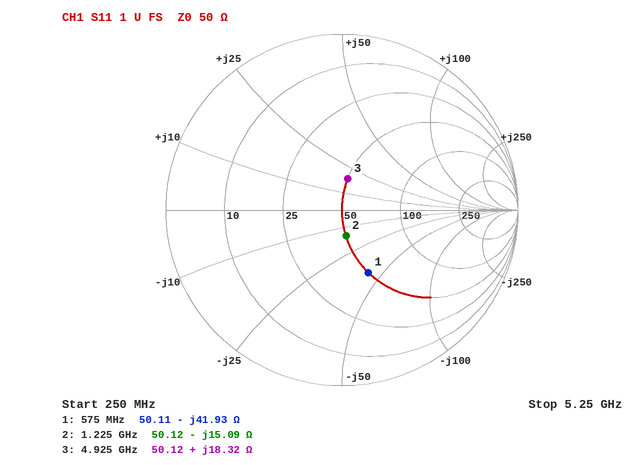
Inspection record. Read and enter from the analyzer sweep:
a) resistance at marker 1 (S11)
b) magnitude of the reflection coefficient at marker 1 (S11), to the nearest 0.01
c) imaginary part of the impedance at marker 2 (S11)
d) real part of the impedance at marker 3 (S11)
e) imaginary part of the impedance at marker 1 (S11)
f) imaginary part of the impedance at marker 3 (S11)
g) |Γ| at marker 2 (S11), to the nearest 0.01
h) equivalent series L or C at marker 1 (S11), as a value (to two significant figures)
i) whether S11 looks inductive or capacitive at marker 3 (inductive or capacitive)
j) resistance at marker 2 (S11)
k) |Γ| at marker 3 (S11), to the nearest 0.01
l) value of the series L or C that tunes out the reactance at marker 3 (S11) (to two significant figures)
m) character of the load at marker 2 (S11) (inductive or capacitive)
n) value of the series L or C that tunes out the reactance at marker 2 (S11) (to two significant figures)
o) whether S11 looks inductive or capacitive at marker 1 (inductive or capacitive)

50.11 Ω
0.39
-15.09 Ω
50.12 Ω
-41.93 Ω
+18.32 Ω
0.15
6.6 pF
inductive
50.12 Ω
0.18
1.8 pF
capacitive
2.0 nH
capacitive
